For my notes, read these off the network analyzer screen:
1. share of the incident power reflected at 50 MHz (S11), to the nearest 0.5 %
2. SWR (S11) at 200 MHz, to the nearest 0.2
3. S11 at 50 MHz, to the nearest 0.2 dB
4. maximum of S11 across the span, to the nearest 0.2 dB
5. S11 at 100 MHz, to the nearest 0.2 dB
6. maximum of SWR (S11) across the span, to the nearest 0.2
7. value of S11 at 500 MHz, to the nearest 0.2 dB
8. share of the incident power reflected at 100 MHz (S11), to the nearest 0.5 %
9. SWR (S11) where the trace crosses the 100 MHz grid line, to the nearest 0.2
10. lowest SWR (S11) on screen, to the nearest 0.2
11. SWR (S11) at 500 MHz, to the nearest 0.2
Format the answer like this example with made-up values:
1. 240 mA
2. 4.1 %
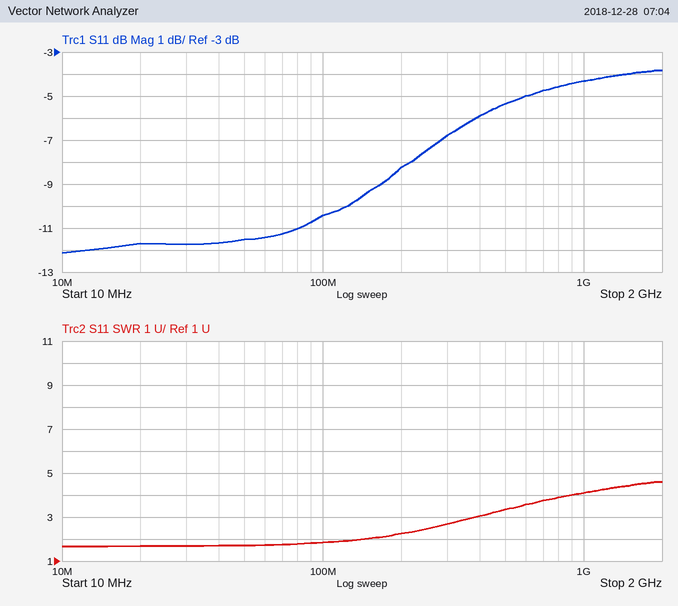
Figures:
1. 7.0 %
2. 2.2
3. -11.6 dB
4. -3.8 dB
5. -10.4 dB
6. 4.6
7. -5.4 dB
8. 9.0 %
9. 1.8
10. 1.6
11. 3.4
